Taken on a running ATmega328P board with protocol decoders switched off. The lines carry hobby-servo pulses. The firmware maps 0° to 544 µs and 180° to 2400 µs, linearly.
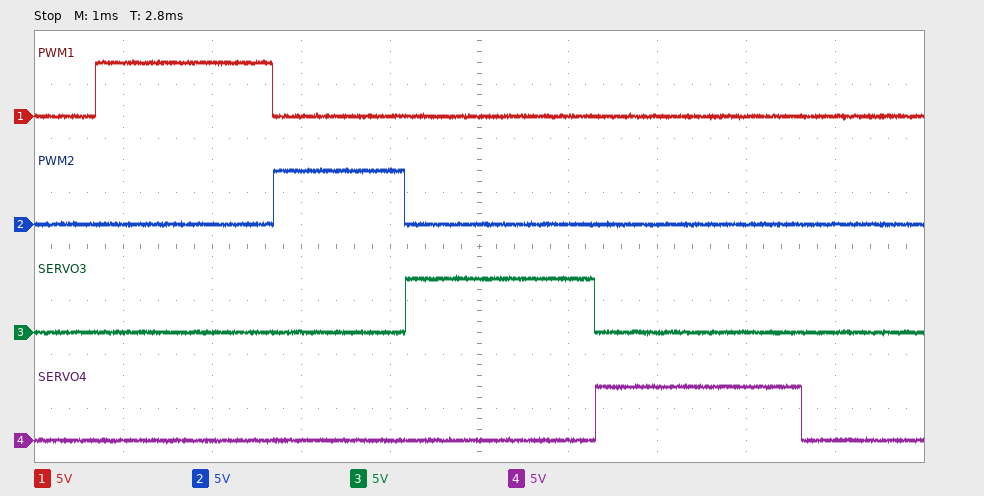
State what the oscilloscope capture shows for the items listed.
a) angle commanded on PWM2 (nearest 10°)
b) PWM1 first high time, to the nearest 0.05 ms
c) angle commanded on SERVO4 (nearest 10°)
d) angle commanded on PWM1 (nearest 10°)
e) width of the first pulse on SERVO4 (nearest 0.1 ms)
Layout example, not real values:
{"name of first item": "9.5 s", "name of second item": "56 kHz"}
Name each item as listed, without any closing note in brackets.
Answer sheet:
{"angle commanded on PWM2": "90°", "PWM1 first high time, to the nearest 0.05 ms": "2.00 ms", "angle commanded on SERVO4": "170°", "angle commanded on PWM1": "140°", "width of the first pulse on SERVO4": "2.3 ms"}
